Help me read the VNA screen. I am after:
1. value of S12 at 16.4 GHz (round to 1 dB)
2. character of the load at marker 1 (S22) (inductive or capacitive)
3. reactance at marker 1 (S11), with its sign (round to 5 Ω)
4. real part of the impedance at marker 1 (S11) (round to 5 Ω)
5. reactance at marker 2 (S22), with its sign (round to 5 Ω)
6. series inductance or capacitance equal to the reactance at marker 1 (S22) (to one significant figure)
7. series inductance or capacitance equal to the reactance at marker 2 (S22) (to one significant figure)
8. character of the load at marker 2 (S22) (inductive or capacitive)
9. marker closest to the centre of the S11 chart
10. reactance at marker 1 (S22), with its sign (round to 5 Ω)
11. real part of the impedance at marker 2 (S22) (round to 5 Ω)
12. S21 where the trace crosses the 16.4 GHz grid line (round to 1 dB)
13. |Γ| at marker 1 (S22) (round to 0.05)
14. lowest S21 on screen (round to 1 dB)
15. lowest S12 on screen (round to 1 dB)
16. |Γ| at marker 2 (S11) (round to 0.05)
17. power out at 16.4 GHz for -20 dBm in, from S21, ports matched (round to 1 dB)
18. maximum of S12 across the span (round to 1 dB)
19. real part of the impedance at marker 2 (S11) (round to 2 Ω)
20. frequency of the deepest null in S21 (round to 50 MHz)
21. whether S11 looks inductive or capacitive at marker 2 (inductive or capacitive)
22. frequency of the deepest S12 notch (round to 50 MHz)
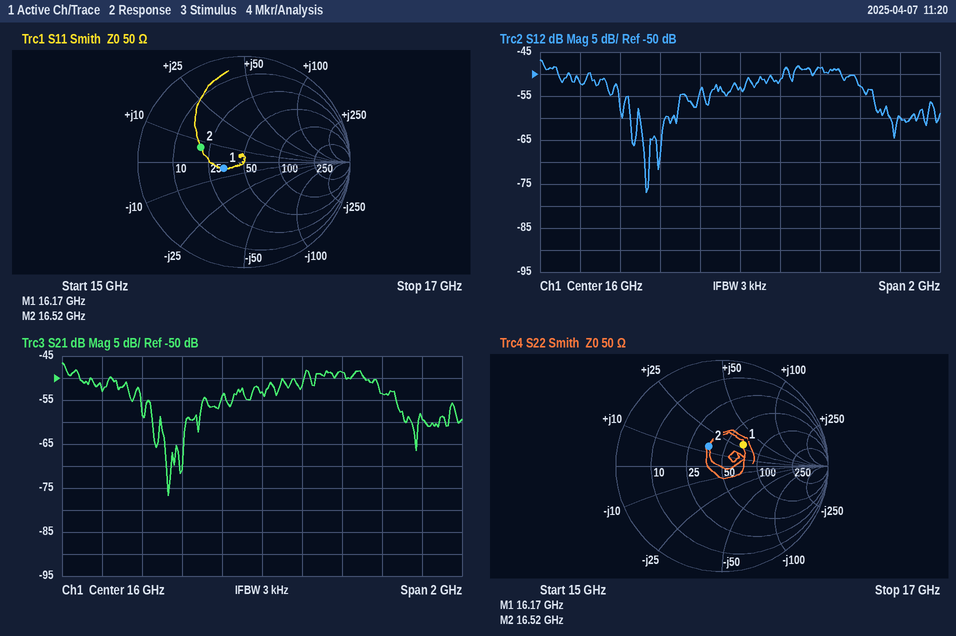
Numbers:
-49 dB
inductive
-5 Ω
35 Ω
+15 Ω
300 pH
100 pH
inductive
marker 1
+30 Ω
35 Ω
-49 dB
0.30
-77 dB
-77 dB
0.45
-69 dBm
-47 dB
20 Ω
15.55 GHz
inductive
15.55 GHz
